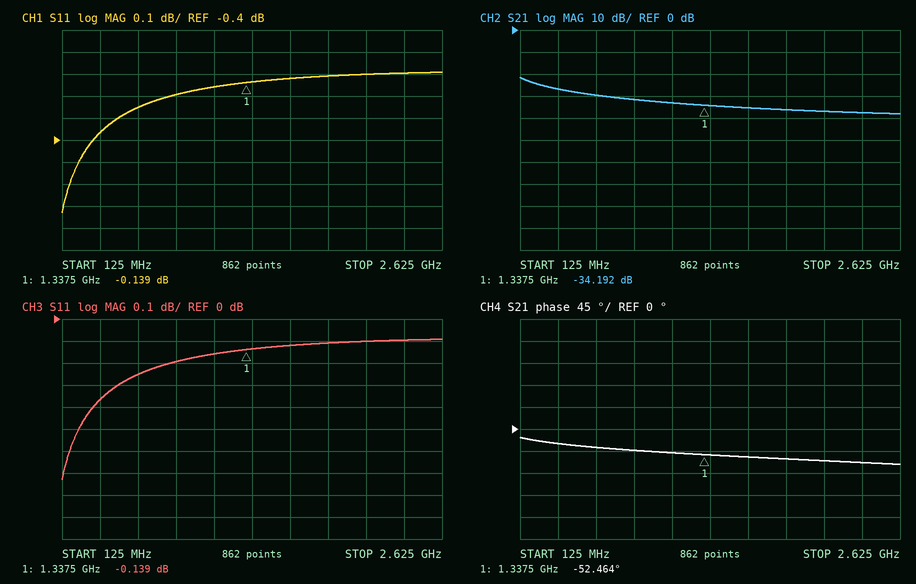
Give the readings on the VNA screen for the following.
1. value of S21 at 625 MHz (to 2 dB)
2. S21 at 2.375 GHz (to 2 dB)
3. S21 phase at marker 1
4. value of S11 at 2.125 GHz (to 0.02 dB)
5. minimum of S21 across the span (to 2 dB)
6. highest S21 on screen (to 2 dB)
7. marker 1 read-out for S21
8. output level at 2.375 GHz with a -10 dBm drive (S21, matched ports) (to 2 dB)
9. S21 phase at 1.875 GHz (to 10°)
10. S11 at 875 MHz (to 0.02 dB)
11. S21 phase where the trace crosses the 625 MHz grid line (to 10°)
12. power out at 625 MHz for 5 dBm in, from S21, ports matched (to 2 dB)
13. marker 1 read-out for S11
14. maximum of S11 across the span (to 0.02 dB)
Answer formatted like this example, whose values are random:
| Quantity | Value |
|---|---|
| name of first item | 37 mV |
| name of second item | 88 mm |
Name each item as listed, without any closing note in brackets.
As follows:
| Quantity | Value |
|---|---|
| value of S21 at 625 MHz | -30 dB |
| S21 at 2.375 GHz | -38 dB |
| S21 phase at marker 1 | -52.464° |
| value of S11 at 2.125 GHz | -0.10 dB |
| minimum of S21 across the span | -38 dB |
| highest S21 on screen | -22 dB |
| marker 1 read-out for S21 | -34.192 dB |
| output level at 2.375 GHz with a -10 dBm drive (S21, matched ports) | -48 dBm |
| S21 phase at 1.875 GHz | -60° |
| S11 at 875 MHz | -0.20 dB |
| S21 phase where the trace crosses the 625 MHz grid line | -40° |
| power out at 625 MHz for 5 dBm in, from S21, ports matched | -24 dBm |
| marker 1 read-out for S11 | -0.139 dB |
| maximum of S11 across the span | -0.10 dB |
